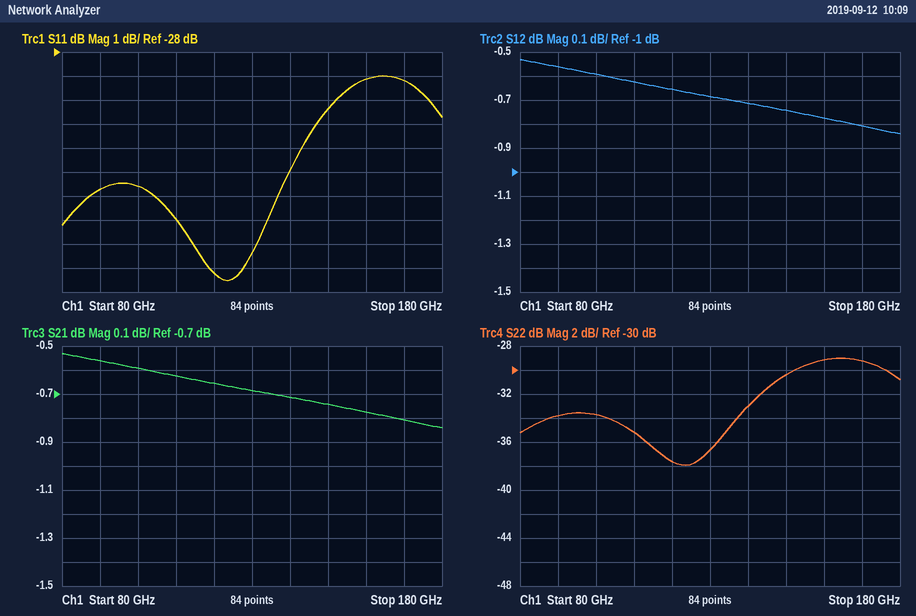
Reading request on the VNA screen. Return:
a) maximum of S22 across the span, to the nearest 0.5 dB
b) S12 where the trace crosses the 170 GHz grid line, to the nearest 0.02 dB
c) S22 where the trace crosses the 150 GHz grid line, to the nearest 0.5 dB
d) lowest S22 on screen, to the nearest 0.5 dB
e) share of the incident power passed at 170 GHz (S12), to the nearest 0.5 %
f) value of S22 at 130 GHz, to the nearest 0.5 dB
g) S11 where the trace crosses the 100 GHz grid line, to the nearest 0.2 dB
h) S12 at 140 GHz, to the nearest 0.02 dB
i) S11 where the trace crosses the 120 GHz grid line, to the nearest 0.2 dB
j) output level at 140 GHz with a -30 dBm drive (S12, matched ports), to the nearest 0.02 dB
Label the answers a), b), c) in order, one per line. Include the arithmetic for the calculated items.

a) -29.0 dB
b) -0.80 dB
c) -30.5 dB
d) -38.0 dB
e) 10^(-0.8/10) ≈ 83.2 %, so 83.0 % to the nearest 0.5 %
f) -36.5 dB
g) -33.6 dB
h) -0.72 dB
i) -37.2 dB
j) -30 dBm + (-0.72 dB) = -30.72 dBm
